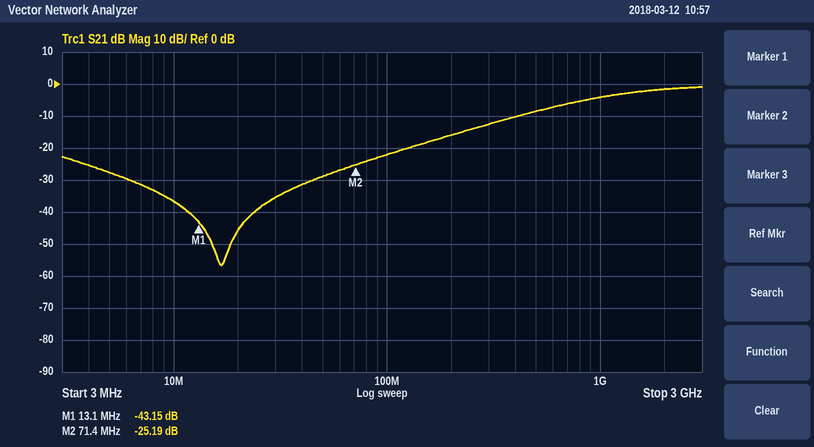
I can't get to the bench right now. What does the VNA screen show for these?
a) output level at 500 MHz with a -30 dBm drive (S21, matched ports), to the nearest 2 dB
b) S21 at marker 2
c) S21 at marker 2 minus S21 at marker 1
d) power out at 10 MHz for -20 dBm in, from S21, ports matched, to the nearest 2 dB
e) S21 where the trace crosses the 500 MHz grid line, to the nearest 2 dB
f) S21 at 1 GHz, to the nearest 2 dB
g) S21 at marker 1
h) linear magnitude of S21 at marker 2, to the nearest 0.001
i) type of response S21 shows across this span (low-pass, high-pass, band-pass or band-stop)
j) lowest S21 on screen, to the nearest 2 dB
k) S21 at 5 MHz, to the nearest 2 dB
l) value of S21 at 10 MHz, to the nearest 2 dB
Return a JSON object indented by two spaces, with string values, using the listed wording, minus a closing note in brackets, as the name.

{
  "output level at 500 MHz with a -30 dBm drive (S21, matched ports), to the nearest 2 dB": "-38 dBm",
  "S21 at marker 2": "-25.19 dB",
  "S21 at marker 2 minus S21 at marker 1": "17.96 dB",
  "power out at 10 MHz for -20 dBm in, from S21, ports matched, to the nearest 2 dB": "-56 dBm",
  "S21 where the trace crosses the 500 MHz grid line, to the nearest 2 dB": "-8 dB",
  "S21 at 1 GHz, to the nearest 2 dB": "-4 dB",
  "S21 at marker 1": "-43.15 dB",
  "linear magnitude of S21 at marker 2, to the nearest 0.001": "0.055",
  "type of response S21 shows across this span": "high-pass",
  "lowest S21 on screen, to the nearest 2 dB": "-56 dB",
  "S21 at 5 MHz, to the nearest 2 dB": "-28 dB",
  "value of S21 at 10 MHz, to the nearest 2 dB": "-36 dB"
}
